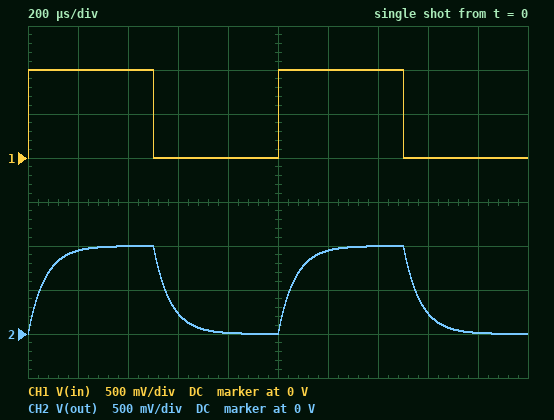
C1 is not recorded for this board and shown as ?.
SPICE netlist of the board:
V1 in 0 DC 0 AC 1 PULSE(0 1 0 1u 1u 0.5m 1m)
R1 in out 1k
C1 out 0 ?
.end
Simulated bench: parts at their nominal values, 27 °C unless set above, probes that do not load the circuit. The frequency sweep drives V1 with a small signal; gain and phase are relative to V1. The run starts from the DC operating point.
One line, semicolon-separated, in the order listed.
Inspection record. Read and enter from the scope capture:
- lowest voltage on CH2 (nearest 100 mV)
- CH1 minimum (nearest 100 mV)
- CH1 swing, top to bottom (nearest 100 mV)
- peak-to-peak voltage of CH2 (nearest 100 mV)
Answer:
0 V; 0 V; 1.0 V; 1.0 V
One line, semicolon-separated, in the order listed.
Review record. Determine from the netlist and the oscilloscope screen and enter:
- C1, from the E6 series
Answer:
68 nF
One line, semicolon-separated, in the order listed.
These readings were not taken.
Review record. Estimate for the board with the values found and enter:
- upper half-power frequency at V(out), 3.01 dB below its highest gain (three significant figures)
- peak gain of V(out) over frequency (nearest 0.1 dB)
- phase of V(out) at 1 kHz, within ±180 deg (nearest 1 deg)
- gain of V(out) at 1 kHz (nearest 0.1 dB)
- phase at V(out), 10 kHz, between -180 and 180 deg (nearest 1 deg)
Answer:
2.34 kHz; 0 dB; -23 deg; -0.7 dB; -77 deg
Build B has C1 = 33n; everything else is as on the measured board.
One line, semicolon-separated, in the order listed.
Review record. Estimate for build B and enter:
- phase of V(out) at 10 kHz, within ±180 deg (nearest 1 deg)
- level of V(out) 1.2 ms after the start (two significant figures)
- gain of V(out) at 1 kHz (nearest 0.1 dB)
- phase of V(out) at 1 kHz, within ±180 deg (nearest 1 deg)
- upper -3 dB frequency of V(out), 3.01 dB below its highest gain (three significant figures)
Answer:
-64 deg; 1.0 V; -0.2 dB; -12 deg; 4.82 kHz
